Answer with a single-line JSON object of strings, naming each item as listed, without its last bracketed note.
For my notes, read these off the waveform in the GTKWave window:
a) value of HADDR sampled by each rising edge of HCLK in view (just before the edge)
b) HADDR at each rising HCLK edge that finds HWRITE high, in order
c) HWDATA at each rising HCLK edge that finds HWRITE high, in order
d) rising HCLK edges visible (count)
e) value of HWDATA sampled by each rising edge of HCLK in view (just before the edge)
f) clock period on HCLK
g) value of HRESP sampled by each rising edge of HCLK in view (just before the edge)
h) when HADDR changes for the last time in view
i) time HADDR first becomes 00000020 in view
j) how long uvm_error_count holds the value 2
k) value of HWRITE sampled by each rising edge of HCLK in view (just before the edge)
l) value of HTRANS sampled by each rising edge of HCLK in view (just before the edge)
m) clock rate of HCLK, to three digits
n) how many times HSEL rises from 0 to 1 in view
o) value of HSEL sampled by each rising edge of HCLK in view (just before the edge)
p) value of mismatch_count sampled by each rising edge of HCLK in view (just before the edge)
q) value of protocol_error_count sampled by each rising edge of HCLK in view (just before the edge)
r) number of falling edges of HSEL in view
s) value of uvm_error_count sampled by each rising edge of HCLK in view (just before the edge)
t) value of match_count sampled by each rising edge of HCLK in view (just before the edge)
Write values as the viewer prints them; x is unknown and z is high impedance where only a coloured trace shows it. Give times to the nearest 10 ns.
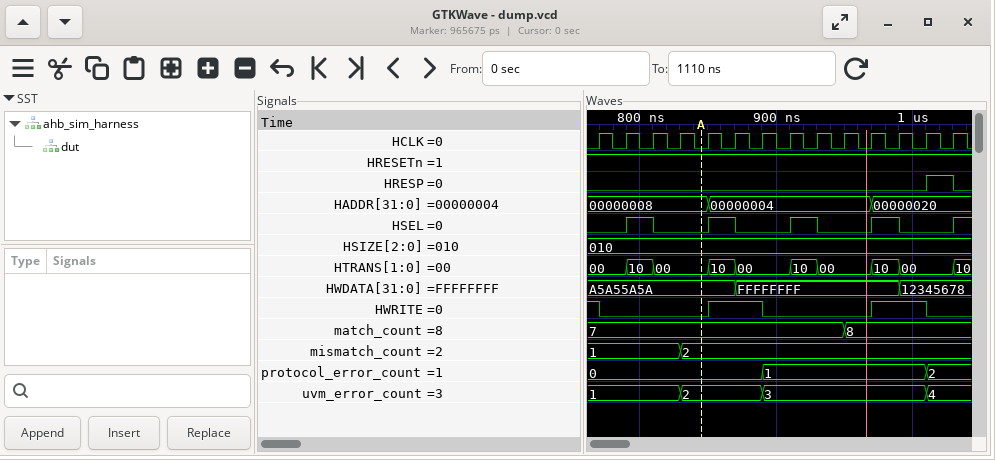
{"value of HADDR sampled by each rising edge of HCLK in view": "00000008, 00000008, 00000008, 00000008, 00000008, 00000004, 00000004, 00000004, 00000004, 00000004, 00000004, 00000020, 00000020, 00000020", "HADDR at each rising HCLK edge that finds HWRITE high, in order": "00000008, 00000004, 00000004, 00000020, 00000020", "HWDATA at each rising HCLK edge that finds HWRITE high, in order": "A5A55A5A, A5A55A5A, FFFFFFFF, FFFFFFFF, 12345678", "rising HCLK edges visible": "14", "value of HWDATA sampled by each rising edge of HCLK in view": "A5A55A5A, A5A55A5A, A5A55A5A, A5A55A5A, A5A55A5A, A5A55A5A, FFFFFFFF, FFFFFFFF, FFFFFFFF, FFFFFFFF, FFFFFFFF, FFFFFFFF, 12345678, 12345678", "clock period on HCLK": "20 ns", "value of HRESP sampled by each rising edge of HCLK in view": "0 0 0 0 0 0 0 0 0 0 0 0 0 1", "when HADDR changes for the last time in view": "970 ns", "time HADDR first becomes 00000020 in view": "970 ns", "how long uvm_error_count holds the value 2": "60 ns", "value of HWRITE sampled by each rising edge of HCLK in view": "1 0 0 0 0 1 1 0 0 0 0 1 1 0", "value of HTRANS sampled by each rising edge of HCLK in view": "00, 00, 10, 00, 00, 10, 00, 00, 10, 00, 00, 10, 00, 00", "clock rate of HCLK, to three digits": "50.0 MHz", "how many times HSEL rises from 0 to 1 in view": "5", "value of HSEL sampled by each rising edge of HCLK in view": "0 0 1 0 0 1 0 0 1 0 0 1 0 0", "value of mismatch_count sampled by each rising edge of HCLK in view": "1, 1, 1, 1, 2, 2, 2, 2, 2, 2, 2, 2, 2, 2", "value of protocol_error_count sampled by each rising edge of HCLK in view": "0, 0, 0, 0, 0, 0, 0, 1, 1, 1, 1, 1, 1, 2", "number of falling edges of HSEL in view": "4", "value of uvm_error_count sampled by each rising edge of HCLK in view": "1, 1, 1, 1, 2, 2, 2, 3, 3, 3, 3, 3, 3, 4", "value of match_count sampled by each rising edge of HCLK in view": "7, 7, 7, 7, 7, 7, 7, 7, 7, 7, 8, 8, 8, 8"}
